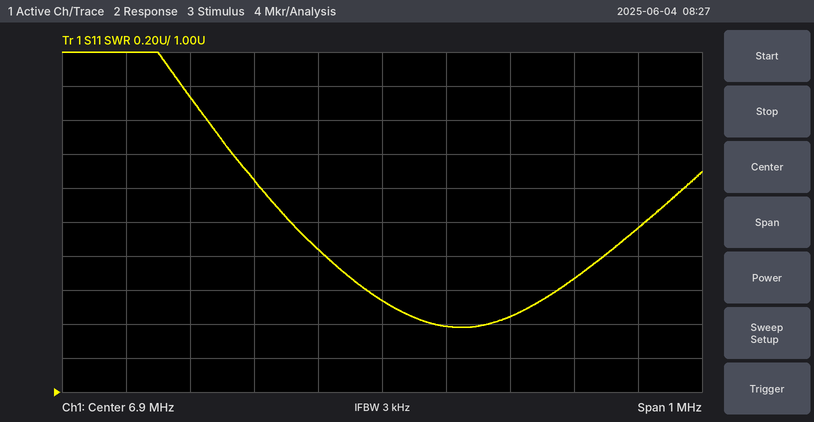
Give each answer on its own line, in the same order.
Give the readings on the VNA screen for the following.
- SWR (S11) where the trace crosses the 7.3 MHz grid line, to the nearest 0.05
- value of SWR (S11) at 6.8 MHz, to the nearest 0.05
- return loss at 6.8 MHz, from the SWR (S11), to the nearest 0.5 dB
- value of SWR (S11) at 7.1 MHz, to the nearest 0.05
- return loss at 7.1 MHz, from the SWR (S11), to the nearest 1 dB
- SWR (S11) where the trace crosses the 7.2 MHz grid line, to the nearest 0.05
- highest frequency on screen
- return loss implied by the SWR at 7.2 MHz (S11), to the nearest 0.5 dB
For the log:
1.95
1.85
10.5 dB
1.45
15 dB
1.65
7.4 MHz
12.0 dB
